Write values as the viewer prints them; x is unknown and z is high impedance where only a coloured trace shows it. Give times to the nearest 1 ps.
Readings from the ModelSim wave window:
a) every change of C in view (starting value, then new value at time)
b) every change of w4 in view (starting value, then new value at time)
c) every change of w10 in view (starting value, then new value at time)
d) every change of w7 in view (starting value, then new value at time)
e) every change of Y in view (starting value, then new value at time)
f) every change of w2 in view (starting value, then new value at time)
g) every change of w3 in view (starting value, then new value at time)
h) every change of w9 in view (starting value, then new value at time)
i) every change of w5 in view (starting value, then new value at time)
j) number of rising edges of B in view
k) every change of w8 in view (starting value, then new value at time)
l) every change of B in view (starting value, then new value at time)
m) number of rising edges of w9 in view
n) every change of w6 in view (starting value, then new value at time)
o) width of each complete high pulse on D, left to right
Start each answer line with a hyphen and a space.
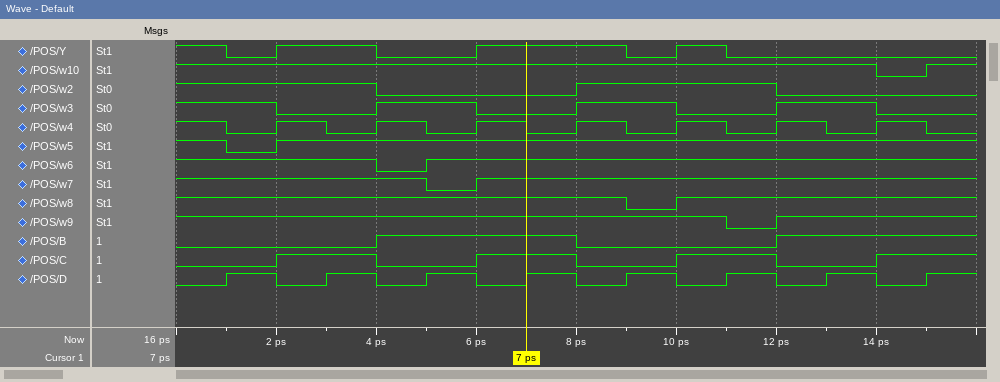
- 0, 1 at 2 ps, 0 at 4 ps, 1 at 6 ps, 0 at 8 ps, 1 at 10 ps, 0 at 12 ps, 1 at 14 ps
- 1, 0 at 1 ps, 1 at 2 ps, 0 at 3 ps, 1 at 4 ps, 0 at 5 ps, 1 at 6 ps, 0 at 7 ps, 1 at 8 ps, 0 at 9 ps, 1 at 10 ps, 0 at 11 ps, 1 at 12 ps, 0 at 13 ps, 1 at 14 ps, 0 at 15 ps
- 1, 0 at 14 ps, 1 at 15 ps
- 1, 0 at 5 ps, 1 at 6 ps
- 1, 0 at 1 ps, 1 at 2 ps, 0 at 4 ps, 1 at 6 ps, 0 at 9 ps, 1 at 10 ps, 0 at 11 ps
- 1, 0 at 4 ps, 1 at 8 ps, 0 at 12 ps
- 1, 0 at 2 ps, 1 at 4 ps, 0 at 6 ps, 1 at 8 ps, 0 at 10 ps, 1 at 12 ps, 0 at 14 ps
- 1, 0 at 11 ps, 1 at 12 ps
- 1, 0 at 1 ps, 1 at 2 ps
- 2
- 1, 0 at 9 ps, 1 at 10 ps
- 0, 1 at 4 ps, 0 at 8 ps, 1 at 12 ps
- 1
- 1, 0 at 4 ps, 1 at 5 ps
- 1 ps, 1 ps, 1 ps, 1 ps, 1 ps, 1 ps, 1 ps
